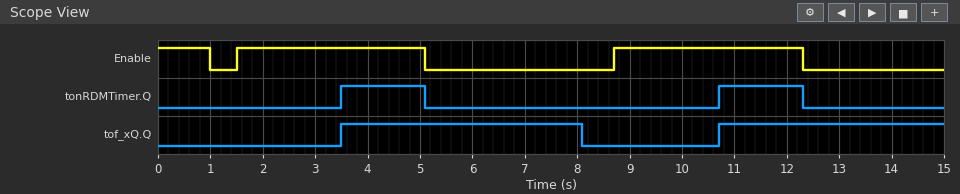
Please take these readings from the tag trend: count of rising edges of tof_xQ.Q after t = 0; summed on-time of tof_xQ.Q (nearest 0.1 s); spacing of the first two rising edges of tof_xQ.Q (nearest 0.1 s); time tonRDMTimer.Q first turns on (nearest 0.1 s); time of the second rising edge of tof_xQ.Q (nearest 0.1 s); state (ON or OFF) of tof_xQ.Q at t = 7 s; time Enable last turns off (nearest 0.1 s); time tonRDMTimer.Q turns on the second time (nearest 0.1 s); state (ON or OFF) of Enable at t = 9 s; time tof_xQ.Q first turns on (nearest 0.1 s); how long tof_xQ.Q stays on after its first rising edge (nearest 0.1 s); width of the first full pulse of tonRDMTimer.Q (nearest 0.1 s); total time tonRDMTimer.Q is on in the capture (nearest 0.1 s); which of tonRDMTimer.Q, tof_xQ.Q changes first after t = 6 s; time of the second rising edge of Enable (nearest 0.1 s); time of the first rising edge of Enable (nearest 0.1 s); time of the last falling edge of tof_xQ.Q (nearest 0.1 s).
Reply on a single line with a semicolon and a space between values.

2; 8.9 s; 7.2 s; 3.5 s; 10.7 s; ON; 12.3 s; 10.7 s; ON; 3.5 s; 4.6 s; 1.6 s; 3.2 s; tof_xQ.Q; 8.7 s; 1.5 s; 8.1 s
